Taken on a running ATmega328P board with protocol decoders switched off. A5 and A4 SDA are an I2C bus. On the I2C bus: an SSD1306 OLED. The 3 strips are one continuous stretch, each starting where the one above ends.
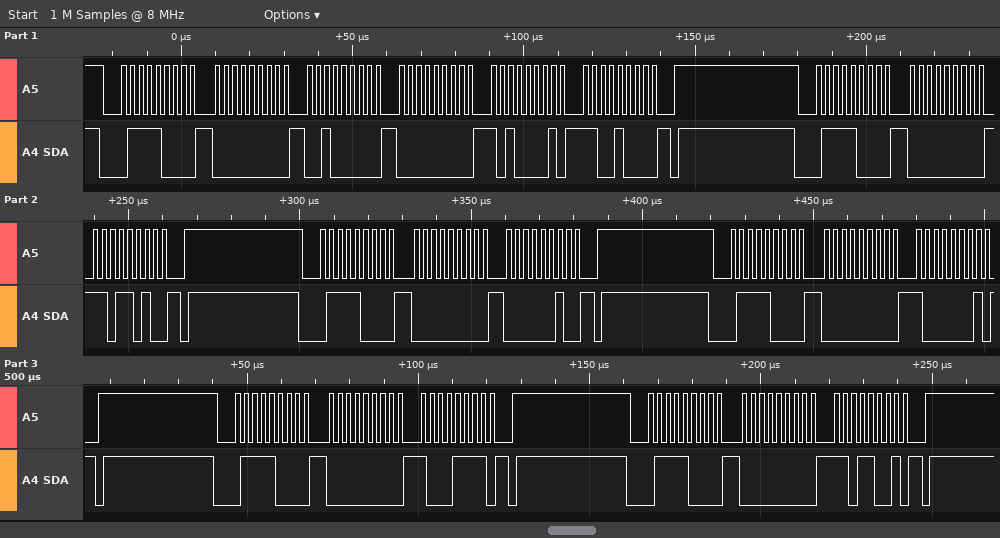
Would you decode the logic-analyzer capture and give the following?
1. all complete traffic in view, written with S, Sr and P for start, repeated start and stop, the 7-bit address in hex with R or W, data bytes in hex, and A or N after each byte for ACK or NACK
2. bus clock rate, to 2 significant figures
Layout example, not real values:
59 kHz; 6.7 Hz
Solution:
S 3CW A 00 A 20 A 00 A A1 A C8 A P S 3CW A 00 A DA A P S 3CW A 00 A 02 A P S 3CW A 00 A 81 A P S 3CW A 00 A 8F A P S 3CW A 00 A D9 A P; 400 kHz
